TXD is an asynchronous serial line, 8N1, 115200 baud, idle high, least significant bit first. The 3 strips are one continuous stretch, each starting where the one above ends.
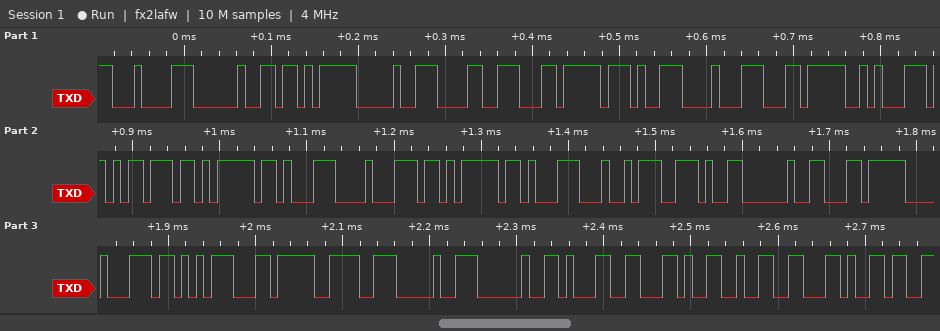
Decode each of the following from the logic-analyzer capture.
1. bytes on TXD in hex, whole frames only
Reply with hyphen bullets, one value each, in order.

- 84 20 EB 90 98 EC 97 88 EC 8A B5 EB 8B 88 EB 8B A4 2E 20 EC 88 AB EC 9E 90 20 31 2C 32 2C
